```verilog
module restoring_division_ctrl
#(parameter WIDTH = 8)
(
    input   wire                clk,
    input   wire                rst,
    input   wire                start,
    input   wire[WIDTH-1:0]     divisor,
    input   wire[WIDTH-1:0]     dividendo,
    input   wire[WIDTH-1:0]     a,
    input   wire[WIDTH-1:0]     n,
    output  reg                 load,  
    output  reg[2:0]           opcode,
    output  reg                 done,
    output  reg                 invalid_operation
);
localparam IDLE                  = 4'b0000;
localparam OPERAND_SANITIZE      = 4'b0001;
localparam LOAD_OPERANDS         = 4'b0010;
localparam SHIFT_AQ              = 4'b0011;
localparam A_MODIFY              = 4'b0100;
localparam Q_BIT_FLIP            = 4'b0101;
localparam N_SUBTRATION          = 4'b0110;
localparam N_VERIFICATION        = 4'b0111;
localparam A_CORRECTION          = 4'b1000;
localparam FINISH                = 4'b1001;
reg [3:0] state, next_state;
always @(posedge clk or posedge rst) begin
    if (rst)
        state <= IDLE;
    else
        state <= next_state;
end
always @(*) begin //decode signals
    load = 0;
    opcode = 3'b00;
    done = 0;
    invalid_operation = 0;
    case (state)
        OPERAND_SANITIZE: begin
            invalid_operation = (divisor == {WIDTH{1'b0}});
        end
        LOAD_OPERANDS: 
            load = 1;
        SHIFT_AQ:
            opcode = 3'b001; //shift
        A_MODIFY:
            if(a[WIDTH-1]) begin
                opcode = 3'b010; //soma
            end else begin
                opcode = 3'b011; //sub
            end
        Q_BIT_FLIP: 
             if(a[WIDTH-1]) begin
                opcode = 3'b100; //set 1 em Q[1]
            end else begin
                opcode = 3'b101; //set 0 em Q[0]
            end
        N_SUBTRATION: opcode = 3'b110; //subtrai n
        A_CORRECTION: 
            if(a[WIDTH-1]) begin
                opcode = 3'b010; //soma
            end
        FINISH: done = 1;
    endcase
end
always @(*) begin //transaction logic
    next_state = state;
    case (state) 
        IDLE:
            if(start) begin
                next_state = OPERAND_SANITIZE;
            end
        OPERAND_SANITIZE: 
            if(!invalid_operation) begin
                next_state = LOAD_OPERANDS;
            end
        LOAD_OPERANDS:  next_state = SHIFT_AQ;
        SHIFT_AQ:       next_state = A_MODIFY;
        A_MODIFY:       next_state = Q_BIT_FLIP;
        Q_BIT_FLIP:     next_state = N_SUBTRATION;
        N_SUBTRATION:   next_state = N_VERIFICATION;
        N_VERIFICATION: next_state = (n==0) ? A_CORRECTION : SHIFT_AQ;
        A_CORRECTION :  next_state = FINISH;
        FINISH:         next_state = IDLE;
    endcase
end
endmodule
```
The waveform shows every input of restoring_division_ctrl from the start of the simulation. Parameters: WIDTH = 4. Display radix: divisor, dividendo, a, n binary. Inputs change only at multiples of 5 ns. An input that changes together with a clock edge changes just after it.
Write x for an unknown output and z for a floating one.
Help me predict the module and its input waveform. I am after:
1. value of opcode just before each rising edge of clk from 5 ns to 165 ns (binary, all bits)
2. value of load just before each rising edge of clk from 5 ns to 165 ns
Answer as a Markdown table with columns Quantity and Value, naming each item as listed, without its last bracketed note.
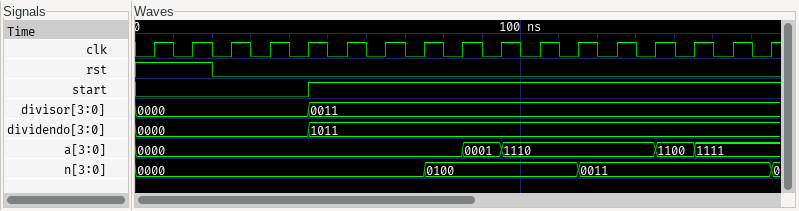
| Quantity | Value |
|---|---|
| value of opcode just before each rising edge of clk from 5 ns to 165 ns | 000, 000, 000, 000, 000, 000, 000, 000, 001, 011, 100, 110, 000, 001, 010, 100, 110 |
| value of load just before each rising edge of clk from 5 ns to 165 ns | 0 0 0 0 0 0 0 1 0 0 0 0 0 0 0 0 0 |
